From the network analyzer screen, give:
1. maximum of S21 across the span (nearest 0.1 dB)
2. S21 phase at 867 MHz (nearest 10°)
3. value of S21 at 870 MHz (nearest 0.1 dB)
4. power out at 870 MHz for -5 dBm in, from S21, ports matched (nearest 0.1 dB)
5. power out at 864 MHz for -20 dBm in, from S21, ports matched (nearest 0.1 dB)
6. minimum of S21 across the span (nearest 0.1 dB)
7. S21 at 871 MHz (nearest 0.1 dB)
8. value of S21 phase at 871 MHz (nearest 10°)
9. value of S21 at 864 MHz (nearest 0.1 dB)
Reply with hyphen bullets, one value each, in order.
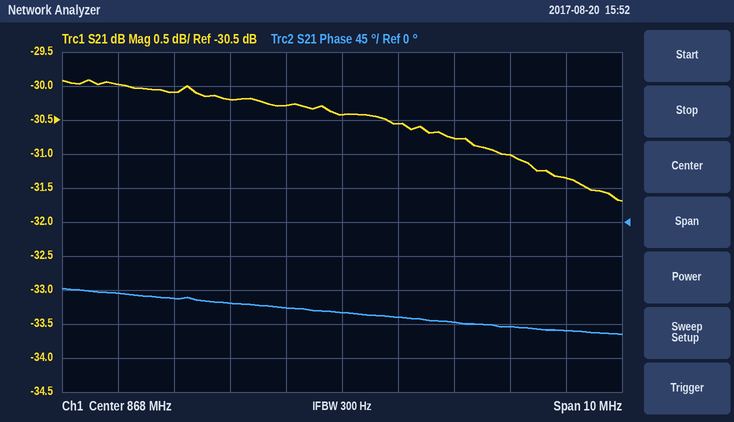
- -29.9 dB
- -110°
- -30.8 dB
- -35.8 dBm
- -50.0 dBm
- -31.7 dB
- -31.0 dB
- -140°
- -30.0 dB
